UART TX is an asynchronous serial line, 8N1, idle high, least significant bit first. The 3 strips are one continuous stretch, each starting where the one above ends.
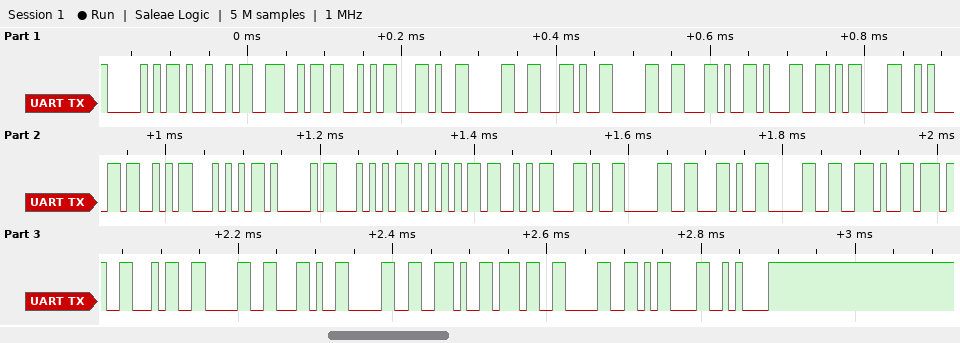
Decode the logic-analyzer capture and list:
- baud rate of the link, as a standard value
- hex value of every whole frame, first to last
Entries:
115200 baud
50 49 4E 53 2C 30 2C 30 2C 31 0D 0A 53 54 41 54 55 53 2C 30 2C 30 2E 37 34 30 2C 30 2E 37 30 0D 0A
